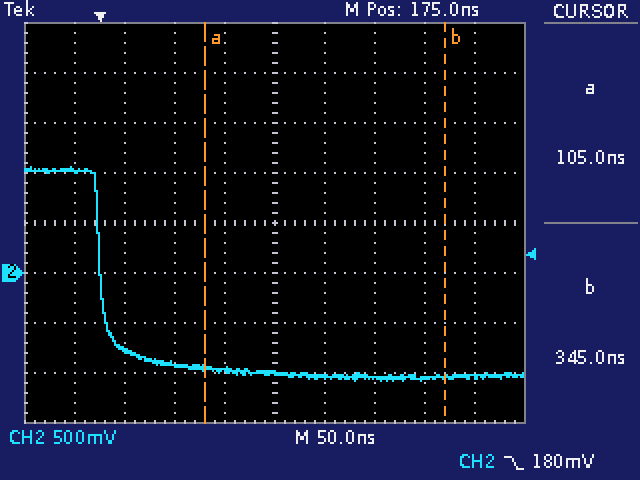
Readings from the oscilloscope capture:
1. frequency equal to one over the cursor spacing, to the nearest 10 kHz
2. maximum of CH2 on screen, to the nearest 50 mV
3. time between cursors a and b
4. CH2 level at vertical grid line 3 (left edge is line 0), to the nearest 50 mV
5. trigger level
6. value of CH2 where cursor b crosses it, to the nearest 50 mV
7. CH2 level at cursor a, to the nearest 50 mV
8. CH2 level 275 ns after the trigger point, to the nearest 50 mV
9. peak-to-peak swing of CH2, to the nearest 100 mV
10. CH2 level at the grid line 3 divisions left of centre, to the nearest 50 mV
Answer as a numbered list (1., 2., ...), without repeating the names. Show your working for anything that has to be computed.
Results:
1. 1 / 240 ns ≈ 4.17 MHz
2. 1.05 V
3. 345 ns − (105 ns) = 240 ns
4. -900 mV
5. 180 mV
6. -1.05 V
7. -950 mV
8. -1.05 V
9. 2.10 V
10. -750 mV
